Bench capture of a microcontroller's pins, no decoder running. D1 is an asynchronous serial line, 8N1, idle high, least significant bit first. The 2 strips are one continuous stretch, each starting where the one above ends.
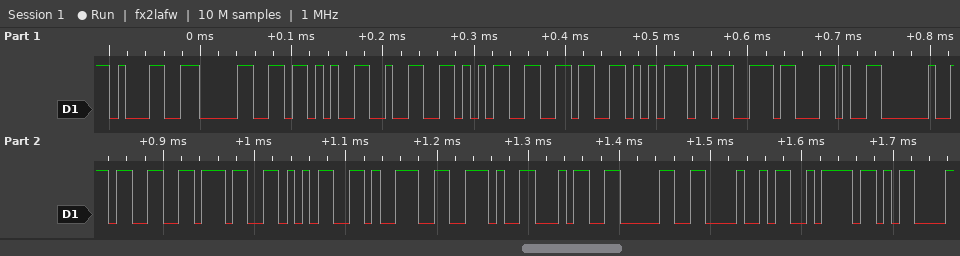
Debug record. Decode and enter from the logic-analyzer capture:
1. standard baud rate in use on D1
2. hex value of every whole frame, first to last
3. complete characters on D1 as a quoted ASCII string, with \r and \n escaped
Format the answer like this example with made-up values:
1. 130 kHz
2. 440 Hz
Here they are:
1. 115200 baud
2. 31 30 2B 32 35 36 75 73 2C 20 33 37 35 39 2E 34 30 48 7A 0D
3. "10+256us, 3759.40Hz\r"
